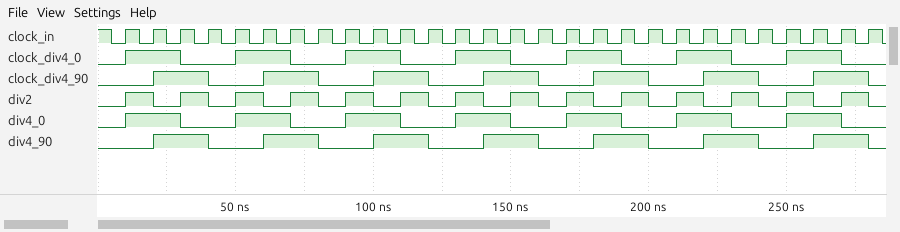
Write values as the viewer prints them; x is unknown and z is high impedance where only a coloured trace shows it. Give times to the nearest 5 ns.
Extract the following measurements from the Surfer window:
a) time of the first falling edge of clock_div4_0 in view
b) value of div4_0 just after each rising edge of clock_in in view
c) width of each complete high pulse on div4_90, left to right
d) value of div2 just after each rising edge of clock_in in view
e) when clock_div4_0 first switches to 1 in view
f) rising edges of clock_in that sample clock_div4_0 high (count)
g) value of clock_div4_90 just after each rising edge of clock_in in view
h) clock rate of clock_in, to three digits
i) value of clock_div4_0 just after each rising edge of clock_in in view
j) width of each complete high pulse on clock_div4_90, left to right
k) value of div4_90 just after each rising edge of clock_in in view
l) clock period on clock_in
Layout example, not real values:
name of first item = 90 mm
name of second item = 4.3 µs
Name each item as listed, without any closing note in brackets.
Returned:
time of the first falling edge of clock_div4_0 in view = 30 ns
value of div4_0 just after each rising edge of clock_in in view = 1 1 0 0 1 1 0 0 1 1 0 0 1 1 0 0 1 1 0 0 1 1 0 0 1 1 0 0
width of each complete high pulse on div4_90, left to right = 20 ns, 20 ns, 20 ns, 20 ns, 20 ns, 20 ns, 20 ns
value of div2 just after each rising edge of clock_in in view = 1 0 1 0 1 0 1 0 1 0 1 0 1 0 1 0 1 0 1 0 1 0 1 0 1 0 1 0
when clock_div4_0 first switches to 1 in view = 10 ns
rising edges of clock_in that sample clock_div4_0 high = 14
value of clock_div4_90 just after each rising edge of clock_in in view = 0 1 1 0 0 1 1 0 0 1 1 0 0 1 1 0 0 1 1 0 0 1 1 0 0 1 1 0
clock rate of clock_in, to three digits = 100 MHz
value of clock_div4_0 just after each rising edge of clock_in in view = 1 1 0 0 1 1 0 0 1 1 0 0 1 1 0 0 1 1 0 0 1 1 0 0 1 1 0 0
width of each complete high pulse on clock_div4_90, left to right = 20 ns, 20 ns, 20 ns, 20 ns, 20 ns, 20 ns, 20 ns
value of div4_90 just after each rising edge of clock_in in view = 0 1 1 0 0 1 1 0 0 1 1 0 0 1 1 0 0 1 1 0 0 1 1 0 0 1 1 0
clock period on clock_in = 10 ns
